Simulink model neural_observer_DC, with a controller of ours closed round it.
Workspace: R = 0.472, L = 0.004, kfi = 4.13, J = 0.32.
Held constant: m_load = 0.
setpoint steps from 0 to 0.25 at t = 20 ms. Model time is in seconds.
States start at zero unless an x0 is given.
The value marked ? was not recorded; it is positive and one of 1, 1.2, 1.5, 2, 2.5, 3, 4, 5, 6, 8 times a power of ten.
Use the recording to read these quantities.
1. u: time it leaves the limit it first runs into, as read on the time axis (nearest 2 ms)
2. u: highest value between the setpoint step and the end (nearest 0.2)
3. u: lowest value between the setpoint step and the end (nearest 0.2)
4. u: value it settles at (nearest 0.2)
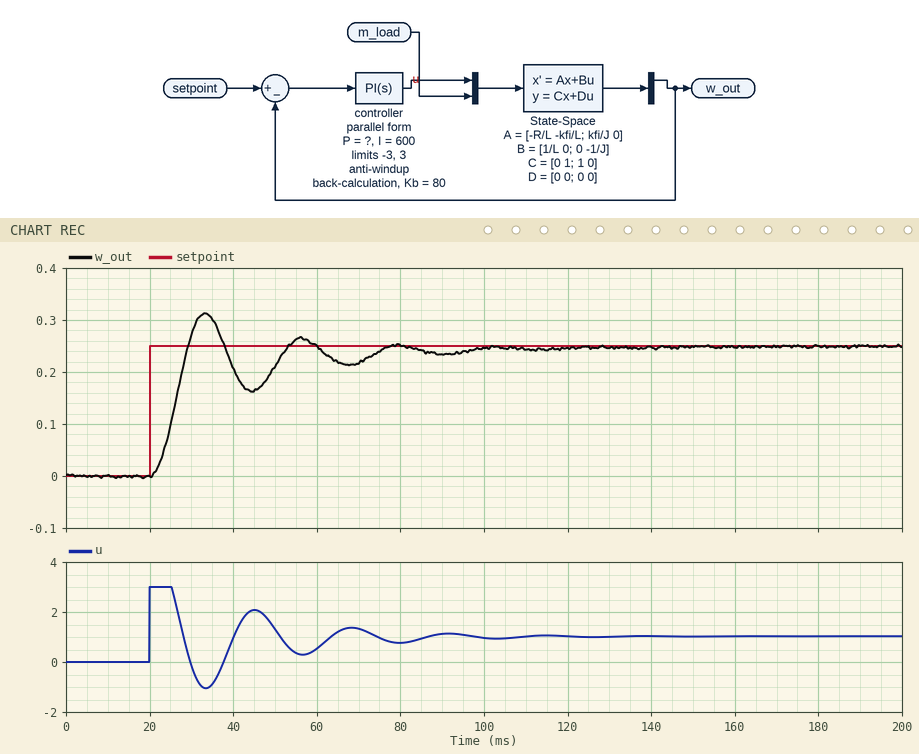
26 ms
3.0
-1.0
1.0
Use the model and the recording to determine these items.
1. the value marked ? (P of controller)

20
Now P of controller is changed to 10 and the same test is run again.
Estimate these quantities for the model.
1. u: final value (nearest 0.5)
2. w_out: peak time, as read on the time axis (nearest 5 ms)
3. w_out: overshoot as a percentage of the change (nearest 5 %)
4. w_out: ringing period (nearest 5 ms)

1.0
35 ms
30 %
30 ms
